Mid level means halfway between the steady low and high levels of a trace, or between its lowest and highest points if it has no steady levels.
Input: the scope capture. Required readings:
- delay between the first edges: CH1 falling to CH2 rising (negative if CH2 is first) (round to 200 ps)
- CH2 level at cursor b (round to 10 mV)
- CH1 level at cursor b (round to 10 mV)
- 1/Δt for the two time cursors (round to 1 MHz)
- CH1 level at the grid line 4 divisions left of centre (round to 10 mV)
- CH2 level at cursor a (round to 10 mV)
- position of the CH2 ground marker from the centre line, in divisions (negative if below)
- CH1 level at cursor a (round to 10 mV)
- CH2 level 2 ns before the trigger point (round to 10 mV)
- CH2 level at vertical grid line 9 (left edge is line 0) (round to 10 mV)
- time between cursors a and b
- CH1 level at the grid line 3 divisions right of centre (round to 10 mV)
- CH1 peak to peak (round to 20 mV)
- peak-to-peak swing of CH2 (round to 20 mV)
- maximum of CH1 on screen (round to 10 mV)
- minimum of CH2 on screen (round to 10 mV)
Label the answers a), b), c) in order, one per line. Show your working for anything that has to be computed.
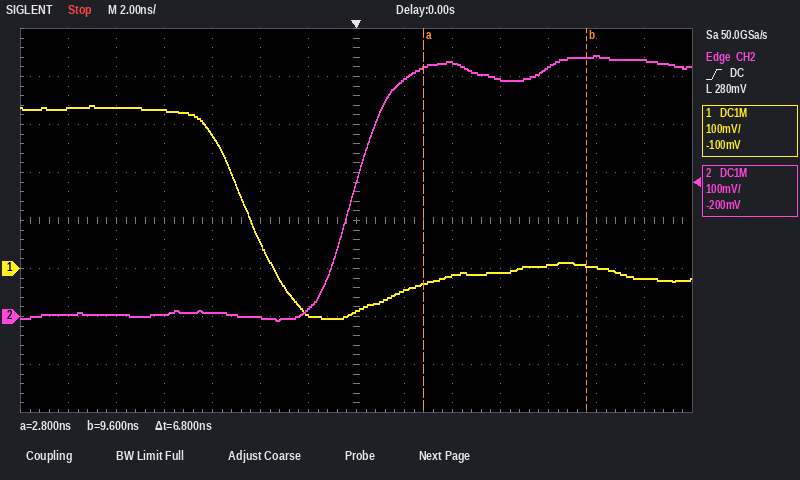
a) +4.4 ns
b) 540 mV
c) 10 mV
d) 1 / 6.8 ns ≈ 147 MHz
e) 330 mV
f) 520 mV
g) -2.0 div
h) -30 mV
i) 20 mV
j) 530 mV
k) 6.8 ns
l) -10 mV
m) 440 mV
n) 560 mV
o) 340 mV
p) -10 mV
